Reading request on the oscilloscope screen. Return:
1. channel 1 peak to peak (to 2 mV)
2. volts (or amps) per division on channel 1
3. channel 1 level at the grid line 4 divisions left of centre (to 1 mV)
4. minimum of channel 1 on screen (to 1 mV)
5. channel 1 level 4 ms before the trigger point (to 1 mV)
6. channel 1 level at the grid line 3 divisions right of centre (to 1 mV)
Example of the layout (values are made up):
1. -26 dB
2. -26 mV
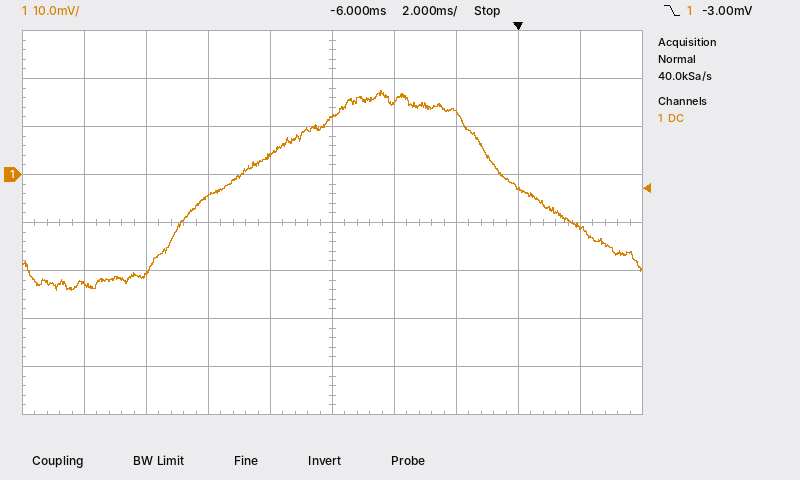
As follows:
1. 42 mV
2. 10 mV
3. -23 mV
4. -24 mV
5. 15 mV
6. -3 mV
